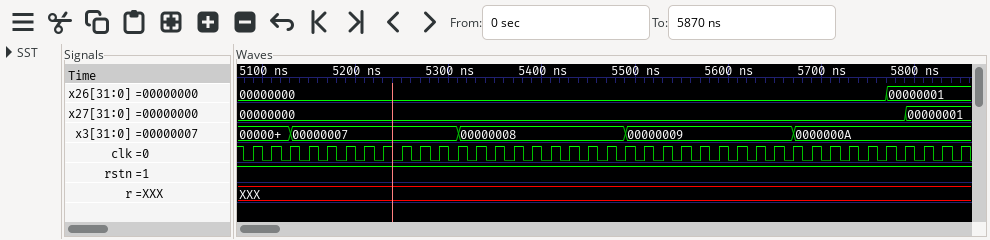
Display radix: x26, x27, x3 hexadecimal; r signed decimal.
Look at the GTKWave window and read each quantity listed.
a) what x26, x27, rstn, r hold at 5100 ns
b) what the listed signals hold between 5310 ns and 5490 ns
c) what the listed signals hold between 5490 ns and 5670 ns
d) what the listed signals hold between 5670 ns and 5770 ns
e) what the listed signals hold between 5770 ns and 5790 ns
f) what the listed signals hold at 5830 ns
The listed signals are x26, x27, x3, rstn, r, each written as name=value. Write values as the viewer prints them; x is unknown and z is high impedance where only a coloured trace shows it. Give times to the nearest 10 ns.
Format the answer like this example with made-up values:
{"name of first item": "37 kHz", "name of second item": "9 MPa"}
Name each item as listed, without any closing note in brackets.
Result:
{"what x26, x27, rstn, r hold at 5100 ns": "x26=00000000, x27=00000000, rstn=1, r=XXX", "what the listed signals hold between 5310 ns and 5490 ns": "x26=00000000, x27=00000000, x3=00000008, rstn=1, r=XXX", "what the listed signals hold between 5490 ns and 5670 ns": "x26=00000000, x27=00000000, x3=00000009, rstn=1, r=XXX", "what the listed signals hold between 5670 ns and 5770 ns": "x26=00000000, x27=00000000, x3=0000000A, rstn=1, r=XXX", "what the listed signals hold between 5770 ns and 5790 ns": "x26=00000001, x27=00000000, x3=0000000A, rstn=1, r=XXX", "what the listed signals hold at 5830 ns": "x26=00000001, x27=00000001, x3=0000000A, rstn=1, r=XXX"}
